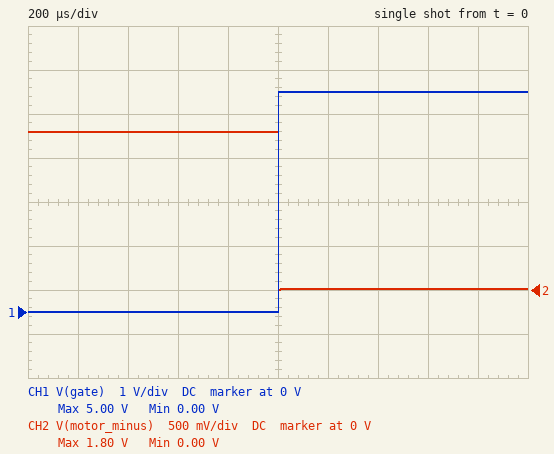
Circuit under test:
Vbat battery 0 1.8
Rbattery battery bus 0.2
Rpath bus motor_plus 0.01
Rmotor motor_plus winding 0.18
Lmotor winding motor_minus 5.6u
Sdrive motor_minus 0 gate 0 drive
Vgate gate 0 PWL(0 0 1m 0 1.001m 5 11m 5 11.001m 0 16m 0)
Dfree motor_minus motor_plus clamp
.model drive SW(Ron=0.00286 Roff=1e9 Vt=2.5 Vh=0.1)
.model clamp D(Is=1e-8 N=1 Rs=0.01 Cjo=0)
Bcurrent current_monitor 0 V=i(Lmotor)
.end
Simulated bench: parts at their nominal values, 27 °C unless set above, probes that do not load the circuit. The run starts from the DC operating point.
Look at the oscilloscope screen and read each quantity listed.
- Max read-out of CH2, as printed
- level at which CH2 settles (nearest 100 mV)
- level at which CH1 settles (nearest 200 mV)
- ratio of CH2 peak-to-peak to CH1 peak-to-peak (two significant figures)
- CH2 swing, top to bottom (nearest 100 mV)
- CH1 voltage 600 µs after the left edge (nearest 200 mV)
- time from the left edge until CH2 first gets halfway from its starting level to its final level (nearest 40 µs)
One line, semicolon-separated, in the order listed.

1.80 V; 0 V; 5.0 V; 0.36; 1.8 V; 0 V; 1.00 ms
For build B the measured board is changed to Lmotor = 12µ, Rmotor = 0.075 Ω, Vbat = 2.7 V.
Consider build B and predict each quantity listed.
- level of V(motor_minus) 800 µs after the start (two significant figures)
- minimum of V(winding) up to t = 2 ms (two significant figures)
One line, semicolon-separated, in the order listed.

2.7 V; 27 mV
